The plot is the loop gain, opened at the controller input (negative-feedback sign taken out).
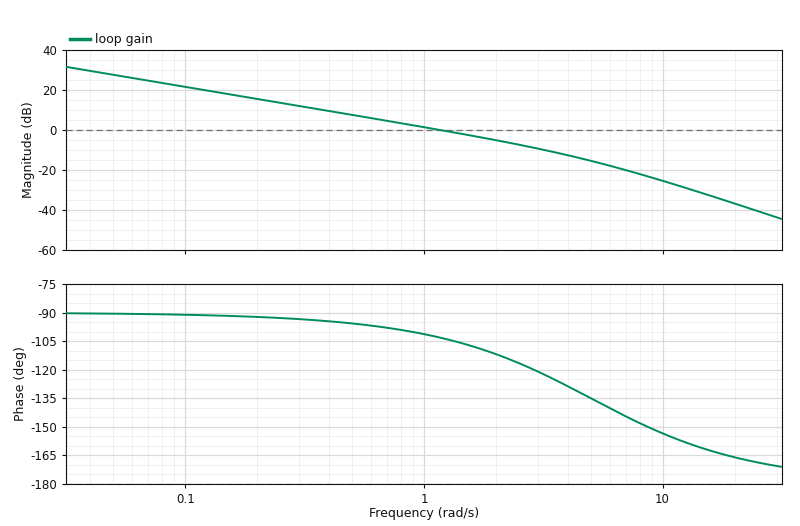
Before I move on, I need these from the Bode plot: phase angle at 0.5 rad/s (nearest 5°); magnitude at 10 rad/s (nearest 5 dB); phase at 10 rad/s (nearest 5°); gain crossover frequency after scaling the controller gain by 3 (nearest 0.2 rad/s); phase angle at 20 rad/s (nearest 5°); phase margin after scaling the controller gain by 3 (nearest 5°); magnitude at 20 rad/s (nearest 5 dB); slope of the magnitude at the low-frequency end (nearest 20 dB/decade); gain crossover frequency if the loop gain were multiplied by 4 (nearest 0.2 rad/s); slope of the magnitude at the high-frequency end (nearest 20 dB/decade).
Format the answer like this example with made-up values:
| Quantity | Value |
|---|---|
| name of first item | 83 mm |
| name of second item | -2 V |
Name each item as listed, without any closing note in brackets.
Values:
| Quantity | Value |
|---|---|
| phase angle at 0.5 rad/s | -95° |
| magnitude at 10 rad/s | -25 dB |
| phase at 10 rad/s | -155° |
| gain crossover frequency after scaling the controller gain by 3 | 3.0 rad/s |
| phase angle at 20 rad/s | -165° |
| phase margin after scaling the controller gain by 3 | 60° |
| magnitude at 20 rad/s | -35 dB |
| slope of the magnitude at the low-frequency end | -20 dB/decade |
| gain crossover frequency if the loop gain were multiplied by 4 | 3.8 rad/s |
| slope of the magnitude at the high-frequency end | -40 dB/decade |
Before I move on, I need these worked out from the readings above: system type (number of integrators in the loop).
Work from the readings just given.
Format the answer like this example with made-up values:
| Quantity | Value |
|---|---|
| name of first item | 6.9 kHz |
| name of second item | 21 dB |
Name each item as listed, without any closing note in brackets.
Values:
| Quantity | Value |
|---|---|
| system type | 1 |
